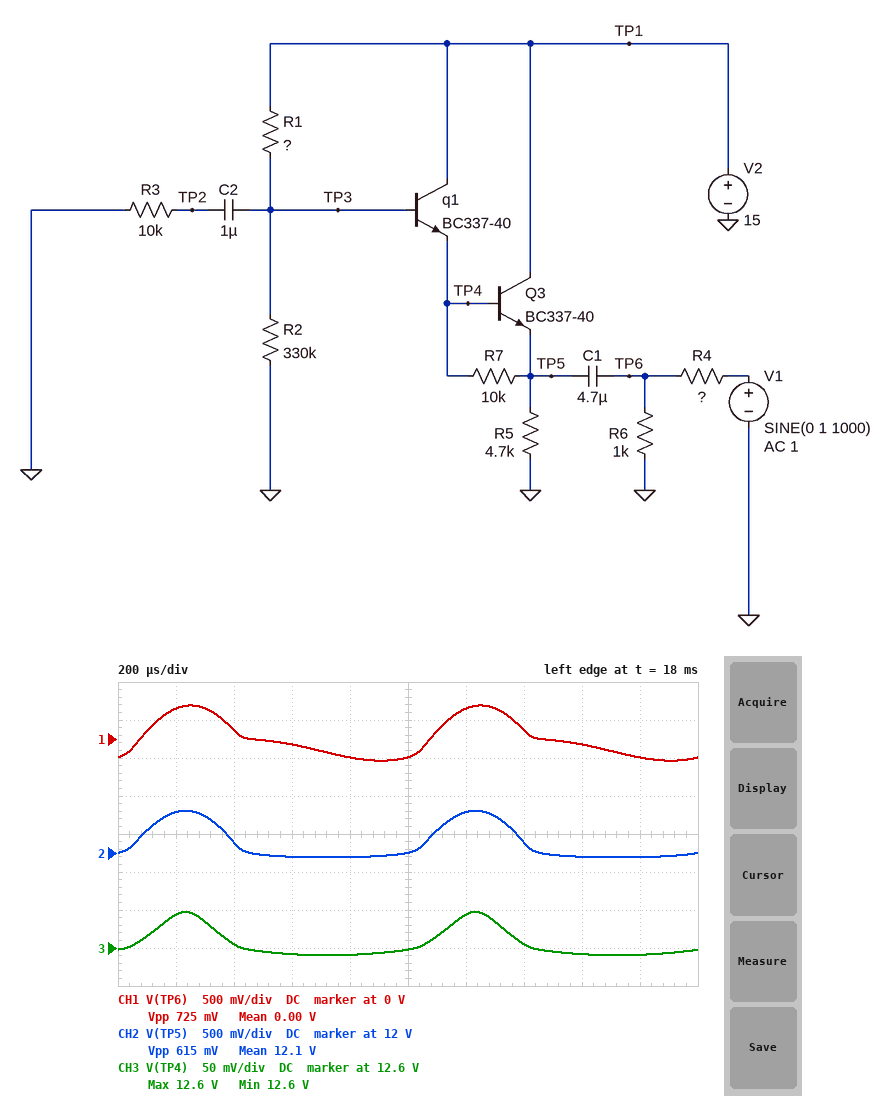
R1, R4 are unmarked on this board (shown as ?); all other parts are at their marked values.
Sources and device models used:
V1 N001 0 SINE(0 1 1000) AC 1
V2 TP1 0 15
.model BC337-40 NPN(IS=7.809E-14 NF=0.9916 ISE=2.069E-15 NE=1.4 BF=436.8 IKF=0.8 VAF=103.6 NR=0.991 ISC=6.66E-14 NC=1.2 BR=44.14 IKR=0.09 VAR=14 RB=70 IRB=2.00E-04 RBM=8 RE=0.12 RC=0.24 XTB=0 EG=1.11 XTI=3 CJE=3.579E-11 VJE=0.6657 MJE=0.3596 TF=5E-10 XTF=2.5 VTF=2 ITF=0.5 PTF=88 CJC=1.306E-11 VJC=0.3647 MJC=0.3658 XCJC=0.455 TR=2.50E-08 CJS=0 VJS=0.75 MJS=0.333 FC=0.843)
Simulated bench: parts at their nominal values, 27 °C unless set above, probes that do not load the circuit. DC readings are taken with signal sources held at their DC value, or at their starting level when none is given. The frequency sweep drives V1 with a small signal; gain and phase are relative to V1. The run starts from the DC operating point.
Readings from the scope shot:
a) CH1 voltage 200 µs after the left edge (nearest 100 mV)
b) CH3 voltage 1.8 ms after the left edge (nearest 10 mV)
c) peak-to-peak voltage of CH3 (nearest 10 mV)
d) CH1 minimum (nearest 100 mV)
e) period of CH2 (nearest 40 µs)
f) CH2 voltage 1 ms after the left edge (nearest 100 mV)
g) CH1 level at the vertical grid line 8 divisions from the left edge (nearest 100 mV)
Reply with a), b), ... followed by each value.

a) 400 mV
b) 12.59 V
c) 60 mV
d) -300 mV
e) 1.00 ms
f) 12.0 V
g) -100 mV
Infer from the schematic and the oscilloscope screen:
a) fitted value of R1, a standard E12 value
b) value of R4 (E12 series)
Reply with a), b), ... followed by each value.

a) 47 kΩ
b) 180 Ω
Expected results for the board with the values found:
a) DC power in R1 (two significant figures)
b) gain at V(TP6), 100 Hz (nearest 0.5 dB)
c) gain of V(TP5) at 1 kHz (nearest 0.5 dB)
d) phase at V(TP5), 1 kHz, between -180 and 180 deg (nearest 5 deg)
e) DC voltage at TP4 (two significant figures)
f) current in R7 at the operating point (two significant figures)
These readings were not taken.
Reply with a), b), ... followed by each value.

a) 75 µW
b) -2.5 dB
c) -24.5 dB
d) 10 deg
e) 13 V
f) 62 µA
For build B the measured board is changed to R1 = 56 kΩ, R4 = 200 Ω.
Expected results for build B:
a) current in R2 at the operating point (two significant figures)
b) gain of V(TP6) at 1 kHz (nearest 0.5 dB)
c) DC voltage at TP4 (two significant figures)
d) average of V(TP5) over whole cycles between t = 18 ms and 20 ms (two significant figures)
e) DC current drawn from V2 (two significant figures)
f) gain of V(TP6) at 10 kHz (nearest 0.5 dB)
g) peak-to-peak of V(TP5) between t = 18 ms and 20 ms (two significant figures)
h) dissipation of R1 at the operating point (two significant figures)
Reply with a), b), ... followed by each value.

a) 39 µA
b) -15.5 dB
c) 12 V
d) 12 V
e) 2.5 mA
f) -24.5 dB
g) 550 mV
h) 85 µW
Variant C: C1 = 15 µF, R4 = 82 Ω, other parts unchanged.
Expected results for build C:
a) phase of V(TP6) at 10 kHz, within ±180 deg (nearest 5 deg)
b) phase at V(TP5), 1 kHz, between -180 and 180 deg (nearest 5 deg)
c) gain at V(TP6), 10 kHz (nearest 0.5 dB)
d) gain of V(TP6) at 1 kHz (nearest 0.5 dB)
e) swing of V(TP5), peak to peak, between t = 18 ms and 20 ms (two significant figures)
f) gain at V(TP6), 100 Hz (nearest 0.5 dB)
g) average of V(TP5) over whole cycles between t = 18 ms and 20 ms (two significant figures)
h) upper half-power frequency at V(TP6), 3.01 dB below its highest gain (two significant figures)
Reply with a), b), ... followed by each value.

a) -5 deg
b) 5 deg
c) -18.0 dB
d) -15.5 dB
e) 1.1 V
f) -3.0 dB
g) 12 V
h) 120 Hz
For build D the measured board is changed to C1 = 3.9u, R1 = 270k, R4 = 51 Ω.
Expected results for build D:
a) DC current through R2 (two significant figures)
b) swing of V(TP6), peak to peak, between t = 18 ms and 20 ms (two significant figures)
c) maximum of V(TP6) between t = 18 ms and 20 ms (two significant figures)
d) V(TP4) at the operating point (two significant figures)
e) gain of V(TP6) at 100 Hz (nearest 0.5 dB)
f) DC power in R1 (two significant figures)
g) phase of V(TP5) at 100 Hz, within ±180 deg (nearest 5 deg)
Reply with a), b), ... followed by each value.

a) 25 µA
b) 1.6 V
c) 860 mV
d) 7.7 V
e) -0.5 dB
f) 170 µW
g) 80 deg
